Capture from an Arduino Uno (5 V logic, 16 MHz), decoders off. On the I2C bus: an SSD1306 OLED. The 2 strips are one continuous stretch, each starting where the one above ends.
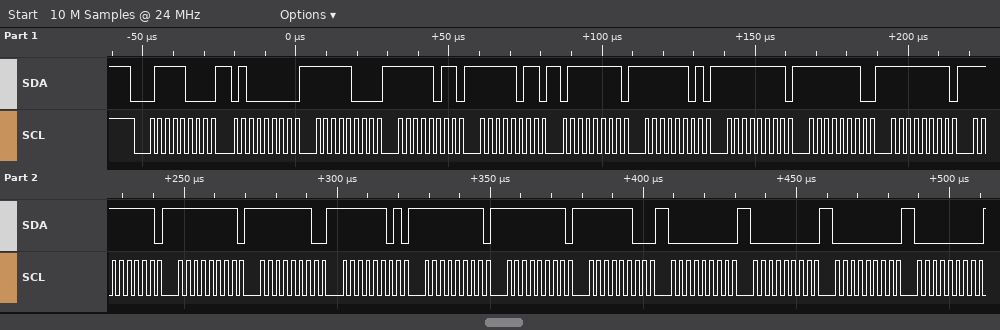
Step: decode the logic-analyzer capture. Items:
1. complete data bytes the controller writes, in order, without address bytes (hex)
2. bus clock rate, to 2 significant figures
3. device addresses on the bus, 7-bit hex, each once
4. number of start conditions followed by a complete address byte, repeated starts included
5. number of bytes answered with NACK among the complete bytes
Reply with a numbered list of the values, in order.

1. 40 F8 FB FB 7F FD FF FE FF FF FF FE FD FF FF FC 00 00 00 00
2. 400 kHz
3. 0x3C
4. 1
5. 0
